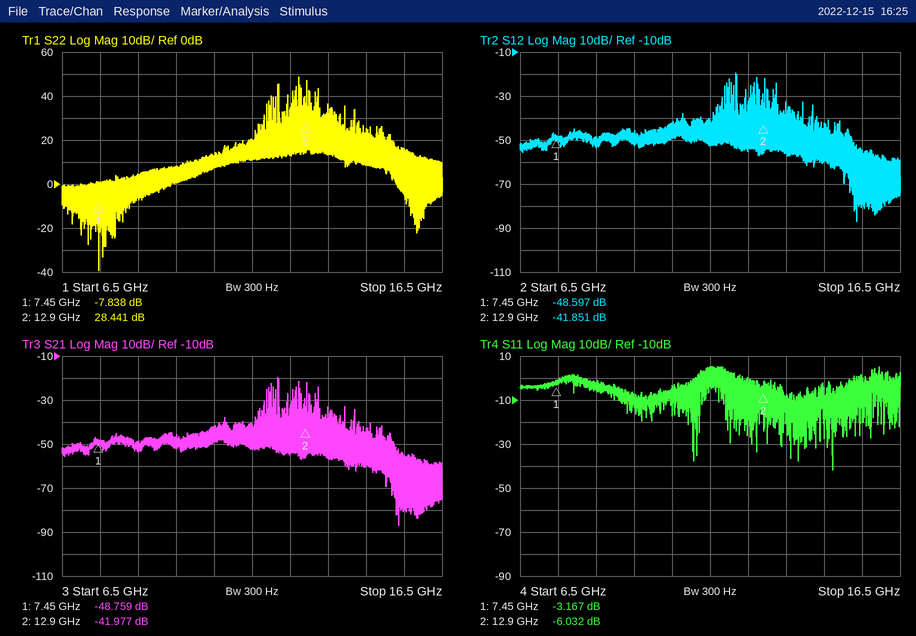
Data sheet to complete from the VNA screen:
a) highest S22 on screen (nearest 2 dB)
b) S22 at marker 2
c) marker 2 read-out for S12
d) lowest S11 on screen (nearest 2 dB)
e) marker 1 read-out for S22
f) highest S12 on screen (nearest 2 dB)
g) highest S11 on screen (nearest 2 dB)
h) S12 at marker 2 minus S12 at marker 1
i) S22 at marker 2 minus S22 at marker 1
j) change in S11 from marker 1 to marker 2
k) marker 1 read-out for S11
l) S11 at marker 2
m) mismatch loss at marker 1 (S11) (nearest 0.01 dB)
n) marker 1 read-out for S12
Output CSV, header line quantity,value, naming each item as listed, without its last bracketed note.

quantity,value
highest S22 on screen,48 dB
S22 at marker 2,28.441 dB
marker 2 read-out for S12,-41.851 dB
lowest S11 on screen,-42 dB
marker 1 read-out for S22,-7.838 dB
highest S12 on screen,-20 dB
highest S11 on screen,6 dB
S12 at marker 2 minus S12 at marker 1,6.746 dB
S22 at marker 2 minus S22 at marker 1,36.279 dB
change in S11 from marker 1 to marker 2,-2.865 dB
marker 1 read-out for S11,-3.167 dB
S11 at marker 2,-6.032 dB
mismatch loss at marker 1 (S11),2.86 dB
marker 1 read-out for S12,-48.597 dB
